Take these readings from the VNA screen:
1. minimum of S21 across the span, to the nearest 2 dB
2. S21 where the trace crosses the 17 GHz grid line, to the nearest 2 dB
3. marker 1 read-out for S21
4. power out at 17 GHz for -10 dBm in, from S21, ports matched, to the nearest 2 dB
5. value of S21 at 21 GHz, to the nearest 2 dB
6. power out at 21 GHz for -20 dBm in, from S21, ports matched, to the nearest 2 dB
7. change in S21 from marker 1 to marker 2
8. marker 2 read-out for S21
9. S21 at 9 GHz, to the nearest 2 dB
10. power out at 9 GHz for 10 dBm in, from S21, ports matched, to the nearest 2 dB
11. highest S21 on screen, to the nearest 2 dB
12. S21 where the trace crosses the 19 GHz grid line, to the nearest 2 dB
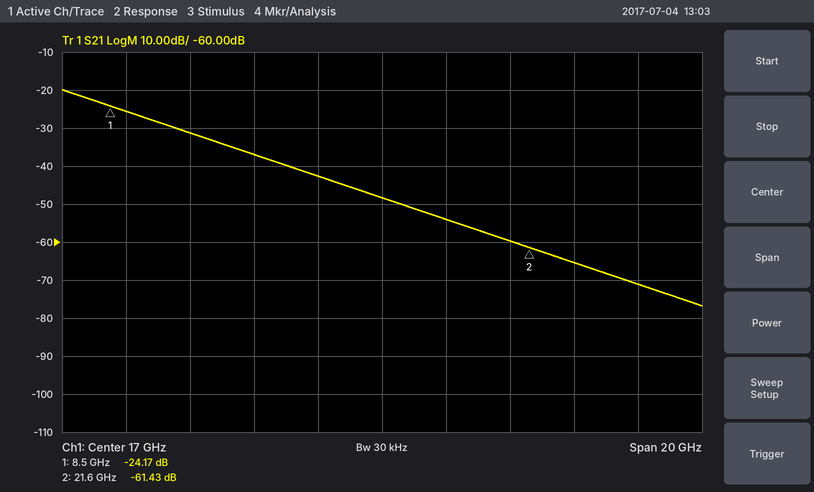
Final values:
-76 dB
-48 dB
-24.17 dB
-58 dBm
-60 dB
-80 dBm
-37.26 dB
-61.43 dB
-26 dB
-16 dBm
-20 dB
-54 dB
